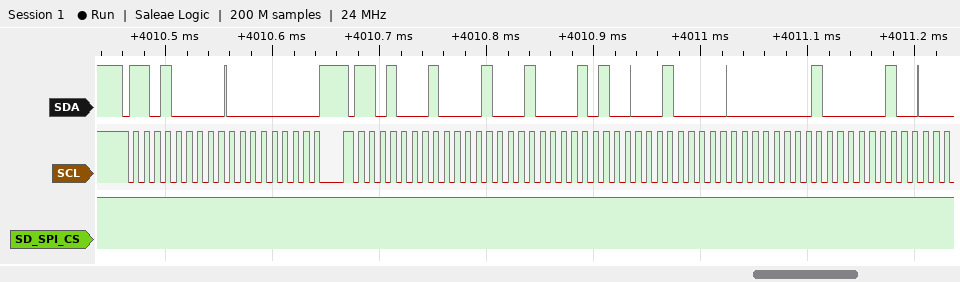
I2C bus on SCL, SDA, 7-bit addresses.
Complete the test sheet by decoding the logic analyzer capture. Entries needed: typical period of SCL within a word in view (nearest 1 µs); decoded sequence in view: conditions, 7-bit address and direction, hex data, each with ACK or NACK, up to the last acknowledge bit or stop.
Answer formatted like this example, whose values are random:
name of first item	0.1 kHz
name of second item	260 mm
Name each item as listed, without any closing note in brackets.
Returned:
typical period of SCL within a word in view	10 µs
decoded sequence in view: conditions, 7-bit address and direction, hex data, each with ACK or NACK, up to the last acknowledge bit or stop	start, address 68 write ACK, 00 ACK, repeated start, address 68 read ACK, 11 ACK, 14 ACK, 20 ACK, 01 ACK, 04 ACK
